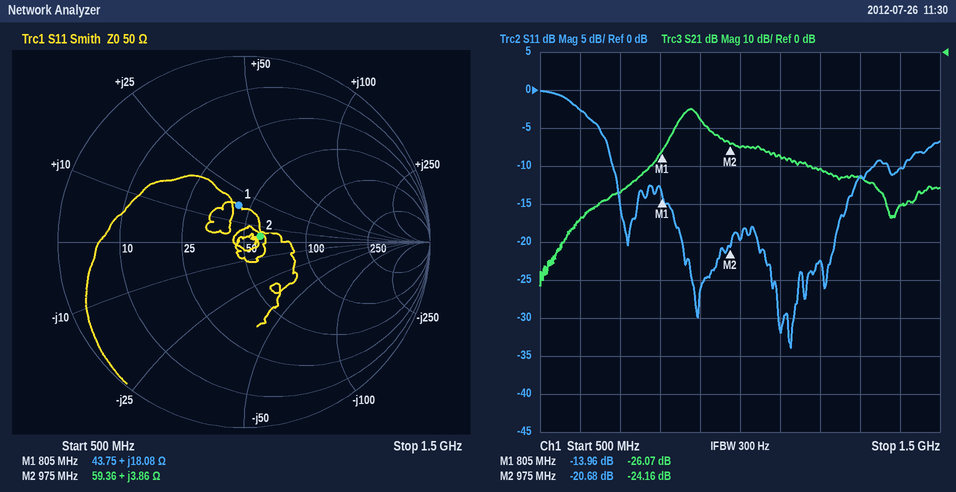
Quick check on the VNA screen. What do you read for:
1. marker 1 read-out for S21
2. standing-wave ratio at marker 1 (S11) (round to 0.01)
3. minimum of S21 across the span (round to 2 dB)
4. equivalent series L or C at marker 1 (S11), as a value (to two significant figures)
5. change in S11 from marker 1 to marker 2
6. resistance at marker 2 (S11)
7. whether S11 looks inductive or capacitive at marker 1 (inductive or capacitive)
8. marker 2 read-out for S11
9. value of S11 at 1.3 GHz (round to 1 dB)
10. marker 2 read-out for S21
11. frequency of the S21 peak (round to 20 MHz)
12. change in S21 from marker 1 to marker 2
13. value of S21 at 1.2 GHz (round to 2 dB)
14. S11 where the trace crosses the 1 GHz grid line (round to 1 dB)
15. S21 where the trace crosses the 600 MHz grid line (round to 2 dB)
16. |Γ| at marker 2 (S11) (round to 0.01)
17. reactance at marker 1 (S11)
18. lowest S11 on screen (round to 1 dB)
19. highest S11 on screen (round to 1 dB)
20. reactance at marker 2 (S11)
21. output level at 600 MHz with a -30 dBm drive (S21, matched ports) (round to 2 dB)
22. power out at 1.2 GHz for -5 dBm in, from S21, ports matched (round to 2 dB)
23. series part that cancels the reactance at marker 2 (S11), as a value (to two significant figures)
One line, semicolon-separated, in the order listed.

-26.07 dB; 1.50; -62 dB; 3.6 nH; -6.72 dB; 59.36 Ω; inductive; -20.68 dB; -11 dB; -24.16 dB; 880 MHz; 1.91 dB; -30 dB; -20 dB; -44 dB; 0.09; +18.08 Ω; -34 dB; 0 dB; +3.86 Ω; -74 dBm; -36 dBm; 42 pF
